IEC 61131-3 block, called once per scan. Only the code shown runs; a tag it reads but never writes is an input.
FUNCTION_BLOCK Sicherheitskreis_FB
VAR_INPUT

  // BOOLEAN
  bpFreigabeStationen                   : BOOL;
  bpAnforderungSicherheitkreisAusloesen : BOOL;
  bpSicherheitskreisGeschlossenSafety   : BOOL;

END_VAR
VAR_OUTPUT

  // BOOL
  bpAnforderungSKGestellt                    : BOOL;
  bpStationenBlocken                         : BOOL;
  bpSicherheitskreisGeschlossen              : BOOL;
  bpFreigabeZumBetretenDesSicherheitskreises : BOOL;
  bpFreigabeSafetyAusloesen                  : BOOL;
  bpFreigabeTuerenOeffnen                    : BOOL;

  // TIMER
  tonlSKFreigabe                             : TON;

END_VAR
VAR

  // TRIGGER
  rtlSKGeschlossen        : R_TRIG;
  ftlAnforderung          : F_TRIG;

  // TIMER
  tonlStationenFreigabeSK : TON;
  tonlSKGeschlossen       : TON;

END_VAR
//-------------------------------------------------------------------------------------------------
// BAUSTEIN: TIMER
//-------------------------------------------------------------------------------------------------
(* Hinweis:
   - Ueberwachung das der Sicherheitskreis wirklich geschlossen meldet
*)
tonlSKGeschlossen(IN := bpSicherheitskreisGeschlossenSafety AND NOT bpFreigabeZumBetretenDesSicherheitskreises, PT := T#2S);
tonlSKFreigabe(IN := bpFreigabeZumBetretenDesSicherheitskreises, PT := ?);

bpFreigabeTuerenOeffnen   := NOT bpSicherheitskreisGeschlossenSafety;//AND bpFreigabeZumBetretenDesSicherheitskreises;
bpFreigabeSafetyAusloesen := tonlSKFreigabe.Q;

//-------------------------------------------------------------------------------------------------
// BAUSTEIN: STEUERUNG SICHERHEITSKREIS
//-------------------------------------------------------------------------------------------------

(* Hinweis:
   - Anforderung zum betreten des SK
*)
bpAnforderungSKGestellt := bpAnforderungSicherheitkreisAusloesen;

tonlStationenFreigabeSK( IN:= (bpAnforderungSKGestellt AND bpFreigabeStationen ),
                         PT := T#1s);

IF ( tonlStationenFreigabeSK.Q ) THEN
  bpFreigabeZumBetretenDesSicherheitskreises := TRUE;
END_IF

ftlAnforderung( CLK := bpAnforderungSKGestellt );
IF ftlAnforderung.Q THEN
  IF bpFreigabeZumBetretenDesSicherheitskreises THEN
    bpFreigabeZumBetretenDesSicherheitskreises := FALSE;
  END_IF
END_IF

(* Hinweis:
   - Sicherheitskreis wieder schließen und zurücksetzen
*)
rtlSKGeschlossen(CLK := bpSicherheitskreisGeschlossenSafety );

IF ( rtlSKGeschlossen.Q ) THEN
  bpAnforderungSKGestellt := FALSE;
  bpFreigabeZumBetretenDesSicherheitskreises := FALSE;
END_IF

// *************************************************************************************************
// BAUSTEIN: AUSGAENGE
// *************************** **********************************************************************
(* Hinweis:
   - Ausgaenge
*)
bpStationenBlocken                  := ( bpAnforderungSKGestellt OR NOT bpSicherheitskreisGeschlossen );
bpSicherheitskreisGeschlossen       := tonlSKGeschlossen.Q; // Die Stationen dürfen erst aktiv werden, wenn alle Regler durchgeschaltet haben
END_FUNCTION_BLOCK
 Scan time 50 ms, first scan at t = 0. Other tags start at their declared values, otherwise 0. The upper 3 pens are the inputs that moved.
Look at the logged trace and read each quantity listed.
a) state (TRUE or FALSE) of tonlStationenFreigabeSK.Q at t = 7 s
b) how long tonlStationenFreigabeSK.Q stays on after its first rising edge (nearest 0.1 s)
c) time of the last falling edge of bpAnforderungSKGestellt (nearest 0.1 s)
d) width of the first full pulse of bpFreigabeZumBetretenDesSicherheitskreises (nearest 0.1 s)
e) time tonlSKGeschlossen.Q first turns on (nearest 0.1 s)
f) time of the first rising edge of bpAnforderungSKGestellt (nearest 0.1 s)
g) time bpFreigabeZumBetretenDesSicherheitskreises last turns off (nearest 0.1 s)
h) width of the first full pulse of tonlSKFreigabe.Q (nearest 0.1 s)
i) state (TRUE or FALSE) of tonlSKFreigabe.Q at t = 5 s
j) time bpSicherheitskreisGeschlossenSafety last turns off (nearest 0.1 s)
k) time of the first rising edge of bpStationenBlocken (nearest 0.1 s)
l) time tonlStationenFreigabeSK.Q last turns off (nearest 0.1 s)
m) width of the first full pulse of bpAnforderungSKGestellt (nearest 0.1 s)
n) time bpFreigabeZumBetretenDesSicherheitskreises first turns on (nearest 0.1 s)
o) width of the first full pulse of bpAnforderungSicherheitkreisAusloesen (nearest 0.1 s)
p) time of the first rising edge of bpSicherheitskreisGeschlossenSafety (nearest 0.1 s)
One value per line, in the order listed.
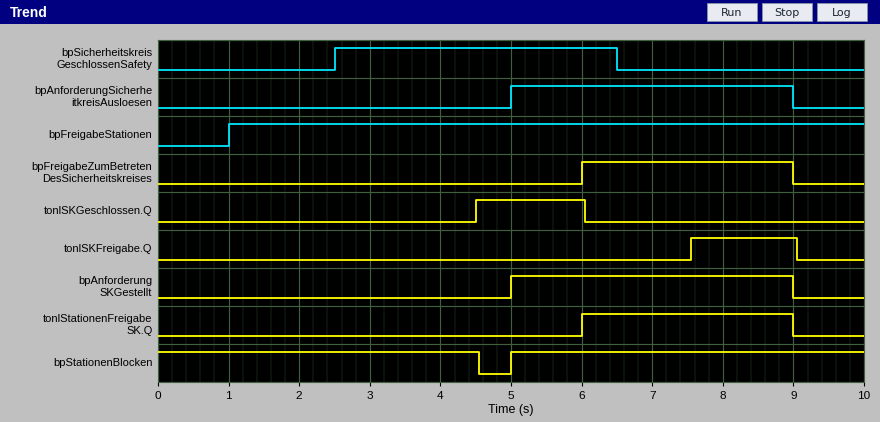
TRUE
3.0 s
9.0 s
3.0 s
4.5 s
5.0 s
9.0 s
1.5 s
FALSE
6.5 s
5.0 s
9.0 s
4.0 s
6.0 s
4.0 s
2.5 s
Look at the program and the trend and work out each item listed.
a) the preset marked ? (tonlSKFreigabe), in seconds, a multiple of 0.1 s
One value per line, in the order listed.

1.5 s
